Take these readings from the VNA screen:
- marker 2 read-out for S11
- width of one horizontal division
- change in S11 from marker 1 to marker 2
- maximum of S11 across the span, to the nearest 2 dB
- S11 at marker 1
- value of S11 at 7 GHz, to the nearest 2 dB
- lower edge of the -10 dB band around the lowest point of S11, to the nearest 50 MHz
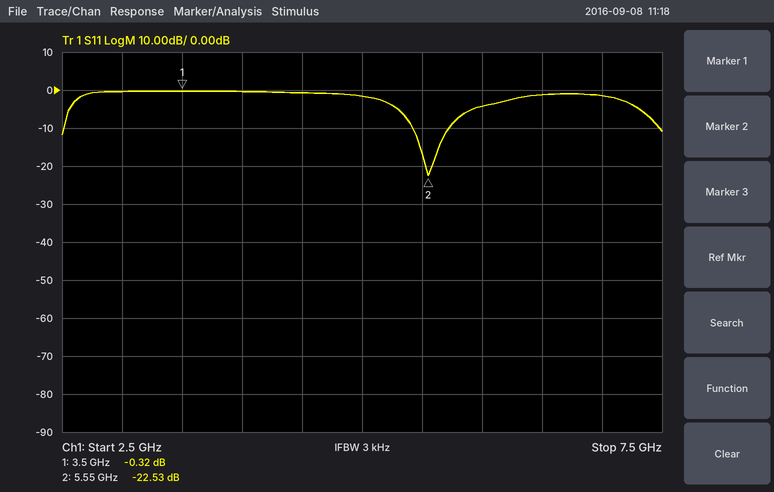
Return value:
-22.53 dB
500 MHz
-22.21 dB
0 dB
-0.32 dB
-2 dB
5.40 GHz
